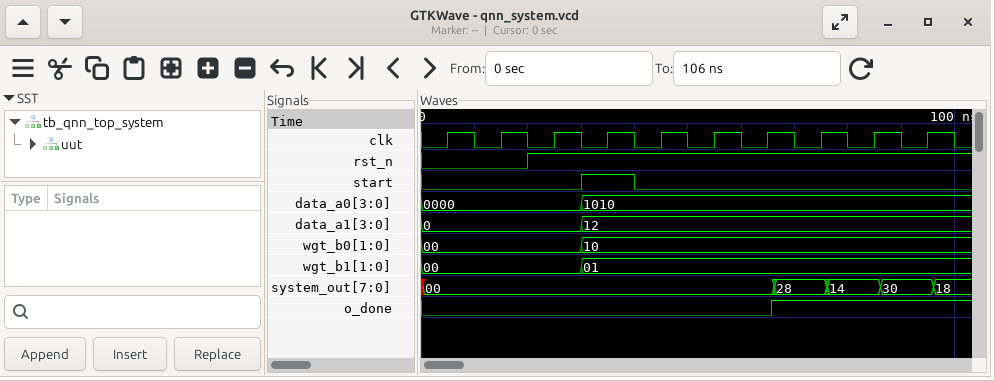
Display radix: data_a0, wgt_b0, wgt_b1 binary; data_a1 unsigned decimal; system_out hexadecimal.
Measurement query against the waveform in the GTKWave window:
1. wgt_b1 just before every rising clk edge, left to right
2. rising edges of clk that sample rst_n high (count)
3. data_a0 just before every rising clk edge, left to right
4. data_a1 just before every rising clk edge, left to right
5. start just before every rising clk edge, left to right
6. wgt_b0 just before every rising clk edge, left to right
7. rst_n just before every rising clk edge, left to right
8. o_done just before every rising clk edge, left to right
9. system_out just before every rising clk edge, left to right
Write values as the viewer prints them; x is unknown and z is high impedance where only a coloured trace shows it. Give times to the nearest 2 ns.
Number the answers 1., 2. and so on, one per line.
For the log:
1. 00, 00, 00, 01, 01, 01, 01, 01, 01, 01
2. 8
3. 0000, 0000, 0000, 1010, 1010, 1010, 1010, 1010, 1010, 1010
4. 0, 0, 0, 12, 12, 12, 12, 12, 12, 12
5. 0 0 0 1 0 0 0 0 0 0
6. 00, 00, 00, 10, 10, 10, 10, 10, 10, 10
7. 0 0 1 1 1 1 1 1 1 1
8. 0 0 0 0 0 0 0 1 1 1
9. 00, 00, 00, 00, 00, 00, 00, 28, 14, 30
